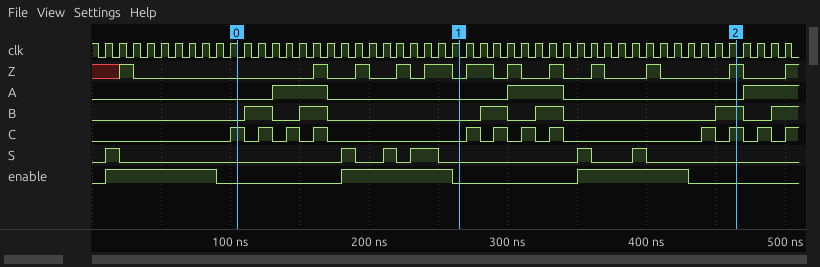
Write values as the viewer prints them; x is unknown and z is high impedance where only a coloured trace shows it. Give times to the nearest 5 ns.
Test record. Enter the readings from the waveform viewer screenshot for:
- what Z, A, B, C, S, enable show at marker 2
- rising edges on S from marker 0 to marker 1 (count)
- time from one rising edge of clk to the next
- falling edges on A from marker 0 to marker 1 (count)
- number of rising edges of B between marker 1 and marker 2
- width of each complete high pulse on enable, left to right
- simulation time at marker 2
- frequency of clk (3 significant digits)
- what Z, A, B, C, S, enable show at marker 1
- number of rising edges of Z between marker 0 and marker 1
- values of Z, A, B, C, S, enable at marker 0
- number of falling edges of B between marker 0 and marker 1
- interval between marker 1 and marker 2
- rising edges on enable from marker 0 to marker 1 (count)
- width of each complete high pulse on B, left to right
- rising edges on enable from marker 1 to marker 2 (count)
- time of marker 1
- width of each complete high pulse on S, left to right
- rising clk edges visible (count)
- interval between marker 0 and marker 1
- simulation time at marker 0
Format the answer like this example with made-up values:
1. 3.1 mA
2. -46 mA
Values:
1. Z=1, A=0, B=1, C=1, S=0, enable=0
2. 3
3. 10 ns
4. 1
5. 3
6. 80 ns, 80 ns, 80 ns
7. 465 ns
8. 100 MHz
9. Z=0, A=0, B=0, C=0, S=0, enable=0
10. 4
11. Z=0, A=0, B=0, C=1, S=0, enable=0
12. 2
13. 200 ns
14. 1
15. 20 ns, 20 ns, 20 ns, 20 ns, 20 ns
16. 1
17. 265 ns
18. 10 ns, 10 ns, 10 ns, 20 ns, 10 ns, 10 ns
19. 50
20. 160 ns
21. 105 ns
